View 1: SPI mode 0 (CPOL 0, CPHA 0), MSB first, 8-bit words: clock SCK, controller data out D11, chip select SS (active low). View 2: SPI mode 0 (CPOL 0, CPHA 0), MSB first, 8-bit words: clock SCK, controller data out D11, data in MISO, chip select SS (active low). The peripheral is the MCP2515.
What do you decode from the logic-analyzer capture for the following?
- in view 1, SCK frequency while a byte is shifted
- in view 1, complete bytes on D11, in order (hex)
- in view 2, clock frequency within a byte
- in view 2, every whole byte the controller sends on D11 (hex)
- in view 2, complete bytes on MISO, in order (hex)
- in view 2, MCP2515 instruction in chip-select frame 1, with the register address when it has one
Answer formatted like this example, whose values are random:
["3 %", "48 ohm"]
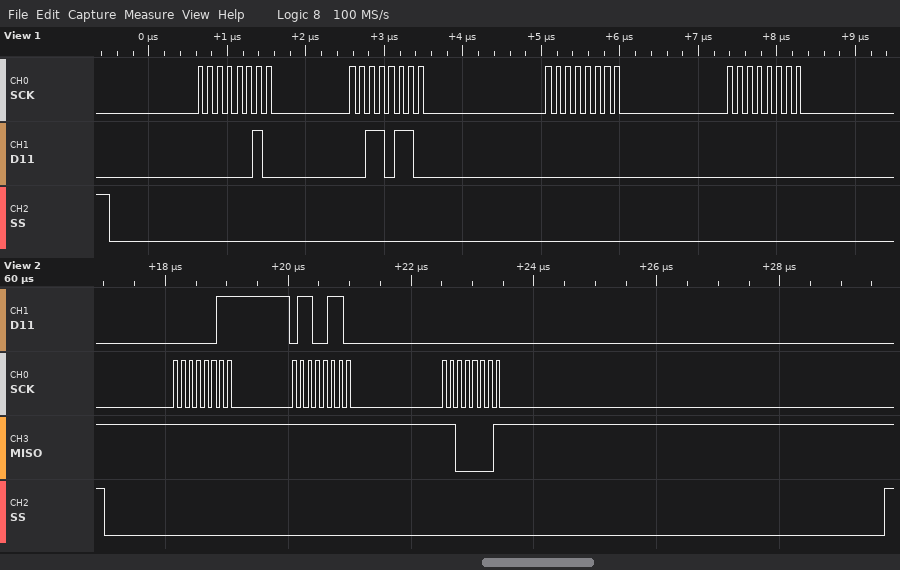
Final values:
["8 MHz", "02 36 00 00", "8 MHz", "0x03 0x66 0x00", "0xFF 0xFF 0xC1", "READ 0x66"]
